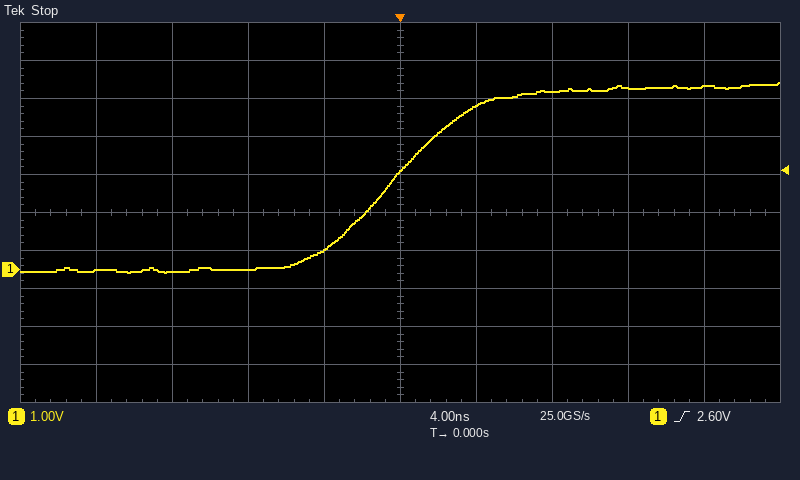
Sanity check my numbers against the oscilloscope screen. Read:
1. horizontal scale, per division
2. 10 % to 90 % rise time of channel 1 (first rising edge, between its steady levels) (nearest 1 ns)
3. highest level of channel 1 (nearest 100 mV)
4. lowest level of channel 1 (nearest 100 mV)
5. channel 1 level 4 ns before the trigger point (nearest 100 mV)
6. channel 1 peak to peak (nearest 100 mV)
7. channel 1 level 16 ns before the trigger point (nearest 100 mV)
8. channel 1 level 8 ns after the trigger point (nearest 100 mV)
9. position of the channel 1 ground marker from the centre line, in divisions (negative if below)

4 ns
8 ns
4.9 V
-100 mV
500 mV
5.0 V
0.0 V
4.7 V
-1.5 div
